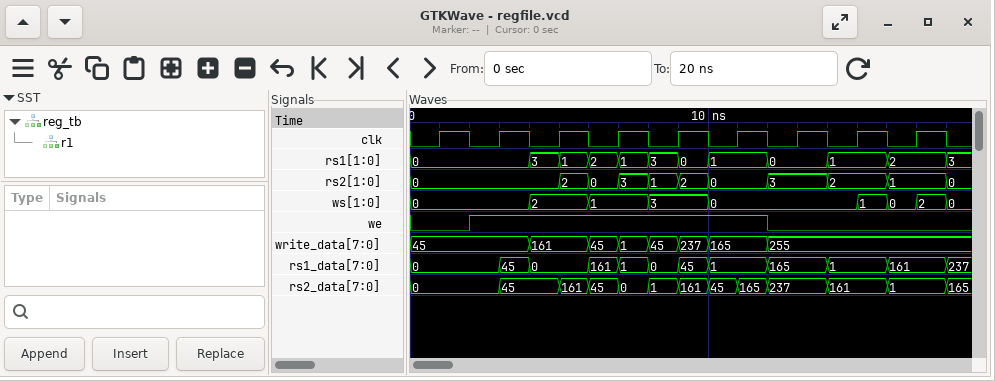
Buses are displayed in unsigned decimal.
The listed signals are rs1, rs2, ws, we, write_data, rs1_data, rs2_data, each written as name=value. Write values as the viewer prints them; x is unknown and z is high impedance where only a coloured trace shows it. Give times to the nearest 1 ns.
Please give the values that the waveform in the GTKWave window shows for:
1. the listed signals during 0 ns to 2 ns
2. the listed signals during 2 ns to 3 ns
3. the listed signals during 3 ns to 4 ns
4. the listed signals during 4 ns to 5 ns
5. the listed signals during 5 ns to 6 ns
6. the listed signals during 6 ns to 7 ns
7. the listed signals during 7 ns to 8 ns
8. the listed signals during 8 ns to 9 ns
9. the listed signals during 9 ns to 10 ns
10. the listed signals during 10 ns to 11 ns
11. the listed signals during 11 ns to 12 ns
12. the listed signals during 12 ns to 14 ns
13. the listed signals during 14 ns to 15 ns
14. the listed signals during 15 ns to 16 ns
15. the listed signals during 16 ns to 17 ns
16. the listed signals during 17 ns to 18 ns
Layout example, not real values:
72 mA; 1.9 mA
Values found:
rs1=0, rs2=0, ws=0, we=0, write_data=45, rs1_data=0, rs2_data=0; rs1=0, rs2=0, ws=0, we=1, write_data=45, rs1_data=0, rs2_data=0; rs1=0, rs2=0, ws=0, we=1, write_data=45, rs1_data=45, rs2_data=45; rs1=3, rs2=0, ws=2, we=1, write_data=161, rs1_data=0, rs2_data=45; rs1=1, rs2=2, ws=2, we=1, write_data=161, rs1_data=0, rs2_data=161; rs1=2, rs2=0, ws=1, we=1, write_data=45, rs1_data=161, rs2_data=45; rs1=1, rs2=3, ws=1, we=1, write_data=1, rs1_data=1, rs2_data=0; rs1=3, rs2=1, ws=3, we=1, write_data=45, rs1_data=0, rs2_data=1; rs1=0, rs2=2, ws=3, we=1, write_data=237, rs1_data=45, rs2_data=161; rs1=1, rs2=0, ws=0, we=1, write_data=165, rs1_data=1, rs2_data=45; rs1=1, rs2=0, ws=0, we=1, write_data=165, rs1_data=1, rs2_data=165; rs1=0, rs2=3, ws=0, we=0, write_data=255, rs1_data=165, rs2_data=237; rs1=1, rs2=2, ws=0, we=0, write_data=255, rs1_data=1, rs2_data=161; rs1=1, rs2=2, ws=1, we=0, write_data=255, rs1_data=1, rs2_data=161; rs1=2, rs2=1, ws=0, we=0, write_data=255, rs1_data=161, rs2_data=1; rs1=2, rs2=1, ws=2, we=0, write_data=255, rs1_data=161, rs2_data=1
